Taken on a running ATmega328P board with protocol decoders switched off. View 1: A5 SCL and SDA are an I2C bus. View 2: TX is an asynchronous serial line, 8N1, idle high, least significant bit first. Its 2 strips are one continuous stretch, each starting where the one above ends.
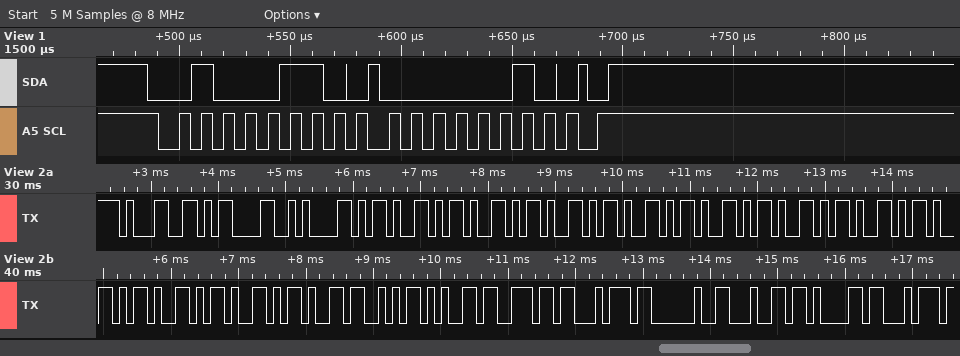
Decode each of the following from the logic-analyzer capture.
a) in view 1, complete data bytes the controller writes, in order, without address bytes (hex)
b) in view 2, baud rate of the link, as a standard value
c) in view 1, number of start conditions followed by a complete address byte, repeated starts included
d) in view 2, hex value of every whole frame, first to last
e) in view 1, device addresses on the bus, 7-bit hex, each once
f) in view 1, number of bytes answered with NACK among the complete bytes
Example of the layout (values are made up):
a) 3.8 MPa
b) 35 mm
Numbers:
a) 02
b) 9600 baud
c) 1
d) 31 0D 0A 2D 2D 2D 2D 2D 2D 2D 2D 2D 2D 2D 53 65 6E 74 20 64 61 74
e) 0x23
f) 0
